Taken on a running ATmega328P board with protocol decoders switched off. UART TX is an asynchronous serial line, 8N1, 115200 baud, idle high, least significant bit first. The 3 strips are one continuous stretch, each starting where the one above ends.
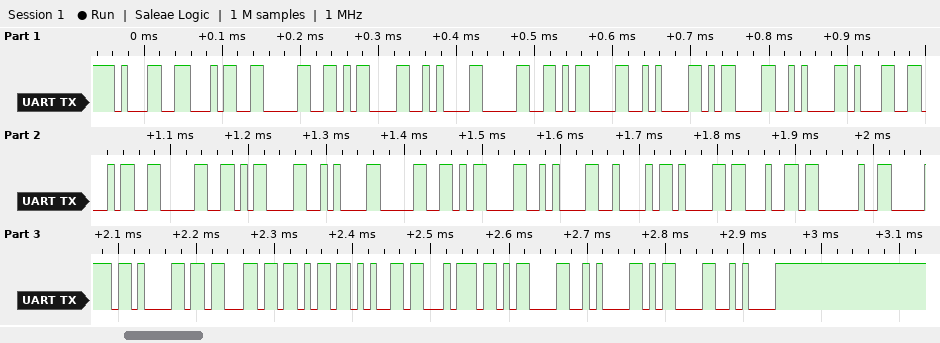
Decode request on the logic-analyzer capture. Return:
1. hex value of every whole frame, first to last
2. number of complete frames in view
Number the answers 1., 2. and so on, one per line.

1. 31 34 30 0D 0A 30 0D 0A 0D 0A 31 34 30 0D 0A 30 0D 0A 42 61 64 20 70 61 63 6B 65 74 0D 0A 0D 0A
2. 32
